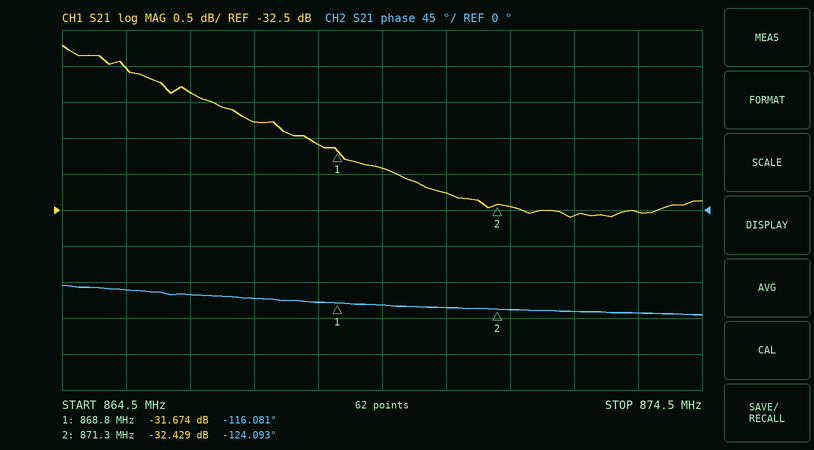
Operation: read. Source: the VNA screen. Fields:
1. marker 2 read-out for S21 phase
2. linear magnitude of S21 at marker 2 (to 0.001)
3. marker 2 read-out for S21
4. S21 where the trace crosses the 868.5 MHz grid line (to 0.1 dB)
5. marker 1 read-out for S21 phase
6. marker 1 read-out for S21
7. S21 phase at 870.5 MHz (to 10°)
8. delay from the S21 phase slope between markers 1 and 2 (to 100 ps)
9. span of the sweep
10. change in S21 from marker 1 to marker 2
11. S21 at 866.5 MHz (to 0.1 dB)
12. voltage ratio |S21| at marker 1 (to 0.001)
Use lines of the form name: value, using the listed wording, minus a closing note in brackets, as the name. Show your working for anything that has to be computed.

marker 2 read-out for S21 phase: -124.093°
linear magnitude of S21 at marker 2: 10^(-32.429/20) ≈ 0.024
marker 2 read-out for S21: -32.429 dB
S21 where the trace crosses the 868.5 MHz grid line: -31.6 dB
marker 1 read-out for S21 phase: -116.081°
marker 1 read-out for S21: -31.674 dB
S21 phase at 870.5 MHz: -120°
delay from the S21 phase slope between markers 1 and 2: −(-124.093° − (-116.081°))/(360° × 2.5 MHz) ≈ 8.9 ns
span of the sweep: 10 MHz
change in S21 from marker 1 to marker 2: -32.429 − (-31.674) = -0.755 dB
S21 at 866.5 MHz: -30.9 dB
voltage ratio |S21| at marker 1: 10^(-31.674/20) ≈ 0.026
